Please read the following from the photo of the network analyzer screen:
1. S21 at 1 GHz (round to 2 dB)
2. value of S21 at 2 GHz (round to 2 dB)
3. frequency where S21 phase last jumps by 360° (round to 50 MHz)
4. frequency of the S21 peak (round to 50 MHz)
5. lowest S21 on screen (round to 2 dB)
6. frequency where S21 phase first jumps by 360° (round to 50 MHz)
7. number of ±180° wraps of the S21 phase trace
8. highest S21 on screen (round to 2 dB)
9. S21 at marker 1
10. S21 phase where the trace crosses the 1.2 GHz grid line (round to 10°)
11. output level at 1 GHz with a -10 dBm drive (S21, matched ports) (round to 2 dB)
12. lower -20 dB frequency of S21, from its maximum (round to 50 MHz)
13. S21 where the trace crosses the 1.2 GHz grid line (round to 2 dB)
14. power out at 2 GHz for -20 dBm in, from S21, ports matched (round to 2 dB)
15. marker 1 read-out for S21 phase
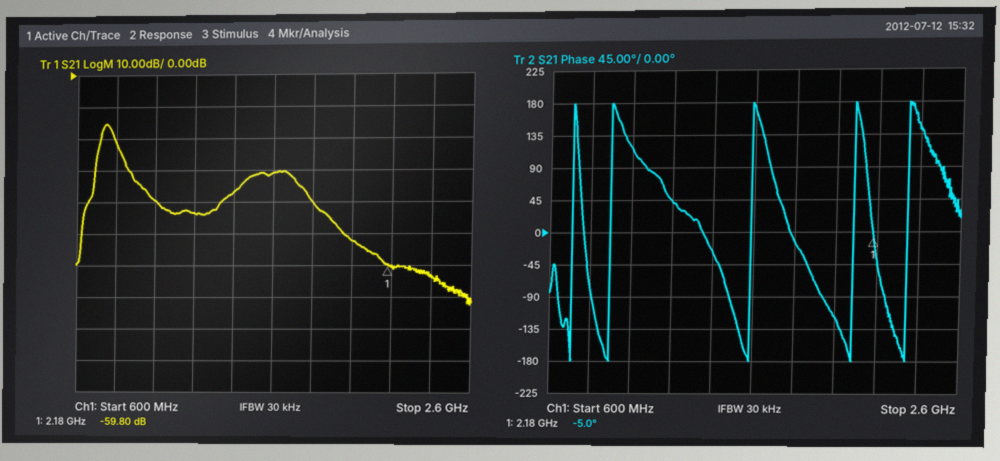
-40 dB
-52 dB
2.35 GHz
750 MHz
-72 dB
700 MHz
5
-16 dB
-59.80 dB
40°
-50 dBm
700 MHz
-44 dB
-72 dBm
-5.0°
